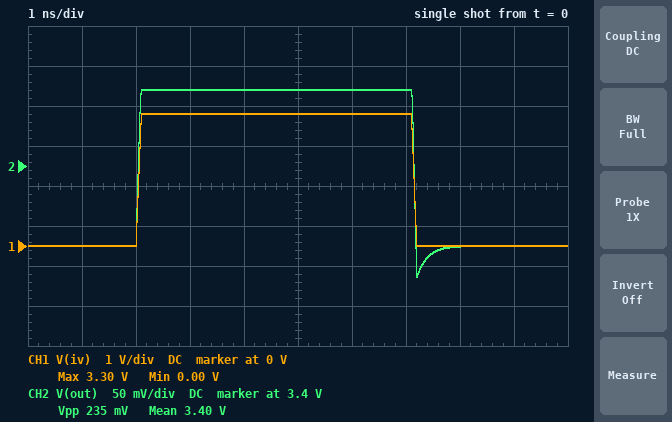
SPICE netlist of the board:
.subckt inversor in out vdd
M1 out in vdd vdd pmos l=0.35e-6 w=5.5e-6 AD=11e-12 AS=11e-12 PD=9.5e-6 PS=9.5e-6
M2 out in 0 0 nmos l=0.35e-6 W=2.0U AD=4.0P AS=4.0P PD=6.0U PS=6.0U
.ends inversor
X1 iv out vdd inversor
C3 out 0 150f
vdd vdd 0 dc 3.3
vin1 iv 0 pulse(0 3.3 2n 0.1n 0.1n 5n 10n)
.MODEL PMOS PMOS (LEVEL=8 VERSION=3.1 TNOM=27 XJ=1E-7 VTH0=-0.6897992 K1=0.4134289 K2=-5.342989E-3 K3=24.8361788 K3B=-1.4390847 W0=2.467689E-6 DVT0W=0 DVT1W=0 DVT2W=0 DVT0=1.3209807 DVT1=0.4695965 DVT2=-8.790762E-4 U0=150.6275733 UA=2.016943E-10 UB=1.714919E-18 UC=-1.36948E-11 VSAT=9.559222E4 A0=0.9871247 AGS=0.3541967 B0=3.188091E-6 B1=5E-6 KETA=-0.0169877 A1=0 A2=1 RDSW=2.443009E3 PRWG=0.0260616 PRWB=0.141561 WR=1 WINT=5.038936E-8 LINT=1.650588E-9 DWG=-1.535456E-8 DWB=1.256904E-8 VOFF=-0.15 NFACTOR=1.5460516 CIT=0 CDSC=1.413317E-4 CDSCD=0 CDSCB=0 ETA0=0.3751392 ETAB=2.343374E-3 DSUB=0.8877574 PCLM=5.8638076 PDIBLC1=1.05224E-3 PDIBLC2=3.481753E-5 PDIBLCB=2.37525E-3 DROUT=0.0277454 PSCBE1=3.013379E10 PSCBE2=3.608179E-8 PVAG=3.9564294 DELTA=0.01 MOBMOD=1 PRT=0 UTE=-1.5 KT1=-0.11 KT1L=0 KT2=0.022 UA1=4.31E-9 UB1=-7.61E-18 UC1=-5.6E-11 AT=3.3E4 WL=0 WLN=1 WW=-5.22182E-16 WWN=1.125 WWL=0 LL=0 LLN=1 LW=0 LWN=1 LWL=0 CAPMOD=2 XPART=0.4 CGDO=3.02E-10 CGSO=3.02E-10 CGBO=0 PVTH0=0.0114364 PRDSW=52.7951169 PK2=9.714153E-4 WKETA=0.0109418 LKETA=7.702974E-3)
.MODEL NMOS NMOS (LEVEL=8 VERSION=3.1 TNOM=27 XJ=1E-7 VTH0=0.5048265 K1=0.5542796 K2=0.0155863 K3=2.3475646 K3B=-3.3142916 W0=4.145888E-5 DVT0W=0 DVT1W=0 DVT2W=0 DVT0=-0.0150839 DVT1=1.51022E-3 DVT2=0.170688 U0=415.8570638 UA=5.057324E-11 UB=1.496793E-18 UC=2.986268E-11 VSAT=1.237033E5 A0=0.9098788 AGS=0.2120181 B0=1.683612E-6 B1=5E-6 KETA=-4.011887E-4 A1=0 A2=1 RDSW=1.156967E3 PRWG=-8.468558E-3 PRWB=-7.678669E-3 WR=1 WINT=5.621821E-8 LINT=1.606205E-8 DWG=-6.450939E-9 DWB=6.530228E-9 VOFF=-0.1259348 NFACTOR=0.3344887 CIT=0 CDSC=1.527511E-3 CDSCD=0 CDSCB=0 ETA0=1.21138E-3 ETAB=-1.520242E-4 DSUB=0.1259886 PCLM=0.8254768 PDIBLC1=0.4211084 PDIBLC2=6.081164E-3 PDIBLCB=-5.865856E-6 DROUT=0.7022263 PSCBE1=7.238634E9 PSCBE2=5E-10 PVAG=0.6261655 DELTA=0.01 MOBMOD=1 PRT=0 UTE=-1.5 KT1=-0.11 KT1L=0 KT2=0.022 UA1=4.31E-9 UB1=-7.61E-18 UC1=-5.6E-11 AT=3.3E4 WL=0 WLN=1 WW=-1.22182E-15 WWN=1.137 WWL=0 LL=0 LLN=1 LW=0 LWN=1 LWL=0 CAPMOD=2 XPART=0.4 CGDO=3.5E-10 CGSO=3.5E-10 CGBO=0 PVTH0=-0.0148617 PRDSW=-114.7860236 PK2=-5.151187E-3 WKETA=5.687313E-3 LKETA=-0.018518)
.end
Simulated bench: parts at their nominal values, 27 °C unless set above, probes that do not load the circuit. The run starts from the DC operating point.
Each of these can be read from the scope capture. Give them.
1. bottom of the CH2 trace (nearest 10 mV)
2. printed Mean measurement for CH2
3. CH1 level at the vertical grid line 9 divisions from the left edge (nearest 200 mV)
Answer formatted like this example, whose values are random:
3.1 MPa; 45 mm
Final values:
3.26 V; 3.40 V; 0 V
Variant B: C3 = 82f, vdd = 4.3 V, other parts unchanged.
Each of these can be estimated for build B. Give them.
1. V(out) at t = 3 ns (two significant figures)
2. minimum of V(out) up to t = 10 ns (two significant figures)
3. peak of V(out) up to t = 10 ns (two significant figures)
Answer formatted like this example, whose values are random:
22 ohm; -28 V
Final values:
4.3 V; 4.0 V; 4.6 V
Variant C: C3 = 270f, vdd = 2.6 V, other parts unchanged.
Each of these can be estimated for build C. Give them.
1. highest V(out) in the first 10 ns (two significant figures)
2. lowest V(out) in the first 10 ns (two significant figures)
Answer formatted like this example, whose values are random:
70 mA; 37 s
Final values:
2.7 V; 2.6 V
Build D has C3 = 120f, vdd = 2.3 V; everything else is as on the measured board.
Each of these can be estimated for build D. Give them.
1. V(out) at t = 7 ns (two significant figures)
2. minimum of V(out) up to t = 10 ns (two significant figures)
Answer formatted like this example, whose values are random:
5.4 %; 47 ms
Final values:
2.5 V; 2.3 V
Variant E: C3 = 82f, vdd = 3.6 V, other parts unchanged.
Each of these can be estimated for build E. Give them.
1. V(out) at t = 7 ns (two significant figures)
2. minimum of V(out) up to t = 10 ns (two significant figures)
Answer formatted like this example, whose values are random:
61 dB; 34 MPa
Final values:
3.9 V; 3.5 V
